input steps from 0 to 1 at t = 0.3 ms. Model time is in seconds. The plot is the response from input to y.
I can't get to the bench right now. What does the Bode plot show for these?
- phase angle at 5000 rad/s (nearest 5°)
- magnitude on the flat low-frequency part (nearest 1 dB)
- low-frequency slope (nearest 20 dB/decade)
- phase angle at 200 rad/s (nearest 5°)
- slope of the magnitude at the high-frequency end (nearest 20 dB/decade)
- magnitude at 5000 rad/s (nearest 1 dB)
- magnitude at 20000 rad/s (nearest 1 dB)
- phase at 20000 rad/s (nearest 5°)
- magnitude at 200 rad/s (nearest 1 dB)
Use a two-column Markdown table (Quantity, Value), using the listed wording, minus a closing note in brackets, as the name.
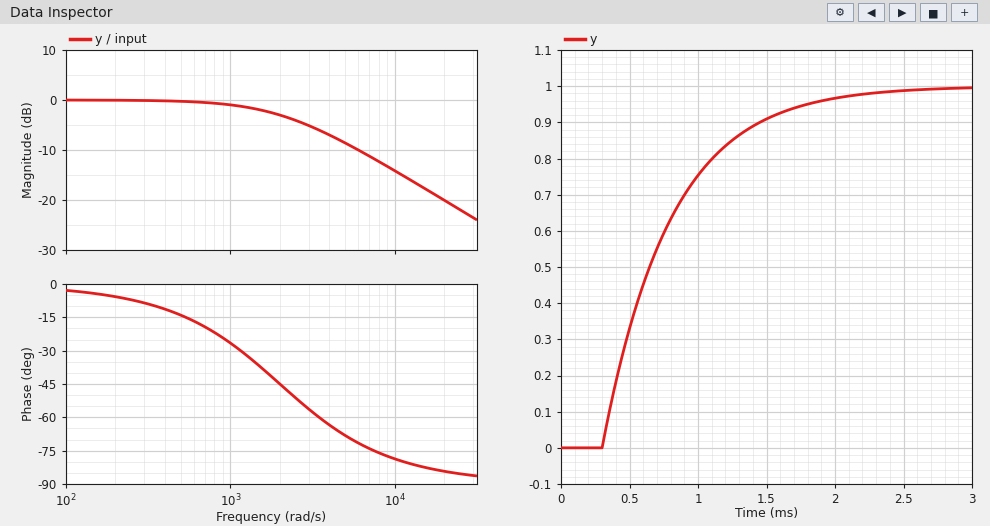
| Quantity | Value |
|---|---|
| phase angle at 5000 rad/s | -70° |
| magnitude on the flat low-frequency part | 0 dB |
| low-frequency slope | 0 dB/decade |
| phase angle at 200 rad/s | -5° |
| slope of the magnitude at the high-frequency end | -20 dB/decade |
| magnitude at 5000 rad/s | -9 dB |
| magnitude at 20000 rad/s | -20 dB |
| phase at 20000 rad/s | -85° |
| magnitude at 200 rad/s | 0 dB |
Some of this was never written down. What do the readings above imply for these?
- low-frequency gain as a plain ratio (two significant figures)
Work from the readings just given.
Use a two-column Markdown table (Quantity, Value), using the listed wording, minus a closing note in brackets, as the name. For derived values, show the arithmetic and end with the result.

| Quantity | Value |
|---|---|
| low-frequency gain as a plain ratio | 10^(0 / 20) = 1.0 |
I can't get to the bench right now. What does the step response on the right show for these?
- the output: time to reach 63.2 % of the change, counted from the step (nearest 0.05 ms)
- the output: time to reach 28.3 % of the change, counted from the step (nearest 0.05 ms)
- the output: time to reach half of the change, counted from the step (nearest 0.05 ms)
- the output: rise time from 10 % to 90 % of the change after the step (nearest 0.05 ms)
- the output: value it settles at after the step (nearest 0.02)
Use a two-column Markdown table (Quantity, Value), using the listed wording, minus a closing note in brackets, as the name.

| Quantity | Value |
|---|---|
| the output: time to reach 63.2 % of the change, counted from the step | 0.50 ms |
| the output: time to reach 28.3 % of the change, counted from the step | 0.15 ms |
| the output: time to reach half of the change, counted from the step | 0.35 ms |
| the output: rise time from 10 % to 90 % of the change after the step | 1.10 ms |
| the output: value it settles at after the step | 1.00 |
